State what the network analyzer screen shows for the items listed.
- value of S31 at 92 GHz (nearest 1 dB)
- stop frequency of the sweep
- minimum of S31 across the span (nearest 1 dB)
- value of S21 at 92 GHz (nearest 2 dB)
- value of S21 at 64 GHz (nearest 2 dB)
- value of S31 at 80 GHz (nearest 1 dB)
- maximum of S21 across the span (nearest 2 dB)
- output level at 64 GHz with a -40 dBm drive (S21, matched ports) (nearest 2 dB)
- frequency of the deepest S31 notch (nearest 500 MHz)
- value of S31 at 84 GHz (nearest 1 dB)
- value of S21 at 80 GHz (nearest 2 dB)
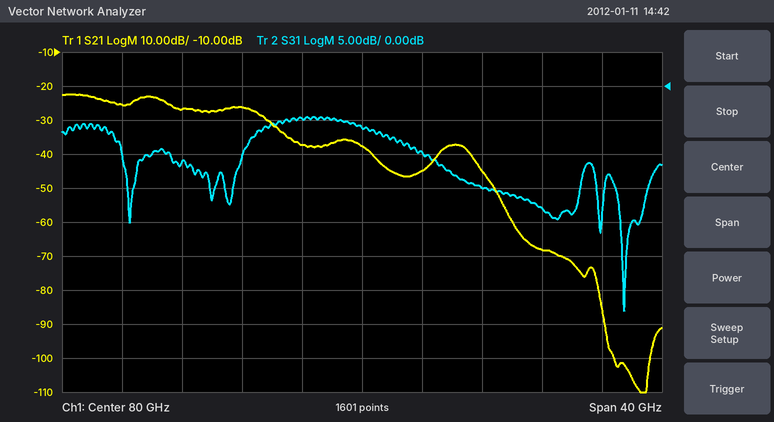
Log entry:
-18 dB
100 GHz
-33 dB
-68 dB
-26 dB
-6 dB
-22 dB
-66 dBm
97.5 GHz
-10 dB
-38 dB
